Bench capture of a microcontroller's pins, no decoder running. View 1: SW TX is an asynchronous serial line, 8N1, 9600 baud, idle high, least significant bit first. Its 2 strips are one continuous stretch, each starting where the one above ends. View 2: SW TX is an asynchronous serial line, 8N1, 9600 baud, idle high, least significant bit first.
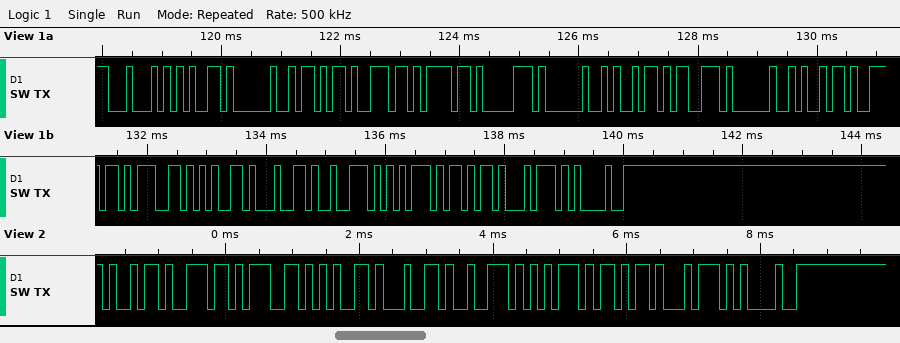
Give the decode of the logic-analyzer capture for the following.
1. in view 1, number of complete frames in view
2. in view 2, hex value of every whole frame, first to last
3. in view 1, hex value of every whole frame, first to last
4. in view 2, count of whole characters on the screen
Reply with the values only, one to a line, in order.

21
0x69 0x6E 0x67 0x65 0x64 0x72 0x75 0x6B 0x74 0x21
44 65 20 6B 6E 6F 70 20 69 73 20 69 6E 67 65 64 72 75 6B 74 21
10
